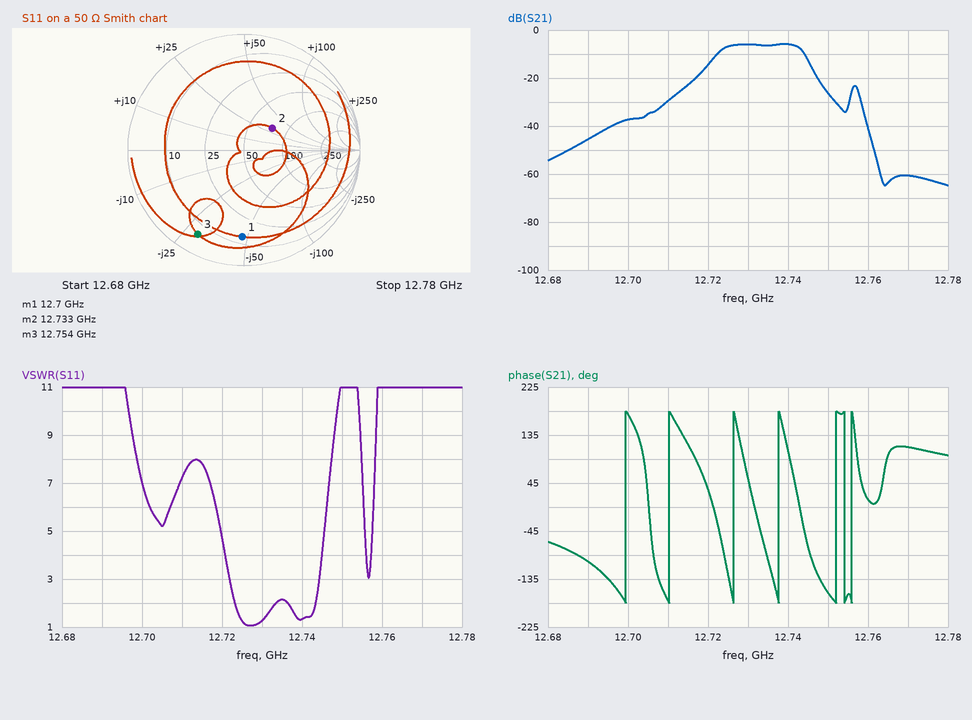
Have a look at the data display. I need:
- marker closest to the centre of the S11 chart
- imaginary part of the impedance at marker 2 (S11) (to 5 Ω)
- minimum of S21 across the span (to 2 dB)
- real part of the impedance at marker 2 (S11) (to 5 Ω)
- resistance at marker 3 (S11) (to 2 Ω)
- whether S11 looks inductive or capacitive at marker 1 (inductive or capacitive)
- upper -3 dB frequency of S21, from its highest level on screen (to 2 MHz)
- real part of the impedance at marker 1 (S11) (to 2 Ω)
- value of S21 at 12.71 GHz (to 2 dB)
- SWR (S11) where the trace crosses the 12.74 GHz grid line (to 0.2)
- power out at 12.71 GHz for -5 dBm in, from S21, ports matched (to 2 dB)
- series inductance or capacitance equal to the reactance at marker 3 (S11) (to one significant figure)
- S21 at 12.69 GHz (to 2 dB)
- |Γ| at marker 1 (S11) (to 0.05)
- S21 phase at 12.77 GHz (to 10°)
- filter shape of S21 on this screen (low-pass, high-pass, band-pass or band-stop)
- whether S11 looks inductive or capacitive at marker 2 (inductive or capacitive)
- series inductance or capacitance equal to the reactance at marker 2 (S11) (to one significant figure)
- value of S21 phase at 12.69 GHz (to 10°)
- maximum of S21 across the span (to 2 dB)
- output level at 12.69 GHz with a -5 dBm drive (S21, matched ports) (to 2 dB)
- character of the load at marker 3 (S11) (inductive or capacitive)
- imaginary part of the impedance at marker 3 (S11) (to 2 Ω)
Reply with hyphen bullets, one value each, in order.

- marker 2
- +30 Ω
- -64 dB
- 75 Ω
- 6 Ω
- capacitive
- 12.744 GHz
- 14 Ω
- -30 dB
- 1.4
- -34 dBm
- 400 fF
- -46 dB
- 0.75
- 110°
- band-pass
- inductive
- 400 pH
- -100°
- -6 dB
- -50 dBm
- capacitive
- -30 Ω
